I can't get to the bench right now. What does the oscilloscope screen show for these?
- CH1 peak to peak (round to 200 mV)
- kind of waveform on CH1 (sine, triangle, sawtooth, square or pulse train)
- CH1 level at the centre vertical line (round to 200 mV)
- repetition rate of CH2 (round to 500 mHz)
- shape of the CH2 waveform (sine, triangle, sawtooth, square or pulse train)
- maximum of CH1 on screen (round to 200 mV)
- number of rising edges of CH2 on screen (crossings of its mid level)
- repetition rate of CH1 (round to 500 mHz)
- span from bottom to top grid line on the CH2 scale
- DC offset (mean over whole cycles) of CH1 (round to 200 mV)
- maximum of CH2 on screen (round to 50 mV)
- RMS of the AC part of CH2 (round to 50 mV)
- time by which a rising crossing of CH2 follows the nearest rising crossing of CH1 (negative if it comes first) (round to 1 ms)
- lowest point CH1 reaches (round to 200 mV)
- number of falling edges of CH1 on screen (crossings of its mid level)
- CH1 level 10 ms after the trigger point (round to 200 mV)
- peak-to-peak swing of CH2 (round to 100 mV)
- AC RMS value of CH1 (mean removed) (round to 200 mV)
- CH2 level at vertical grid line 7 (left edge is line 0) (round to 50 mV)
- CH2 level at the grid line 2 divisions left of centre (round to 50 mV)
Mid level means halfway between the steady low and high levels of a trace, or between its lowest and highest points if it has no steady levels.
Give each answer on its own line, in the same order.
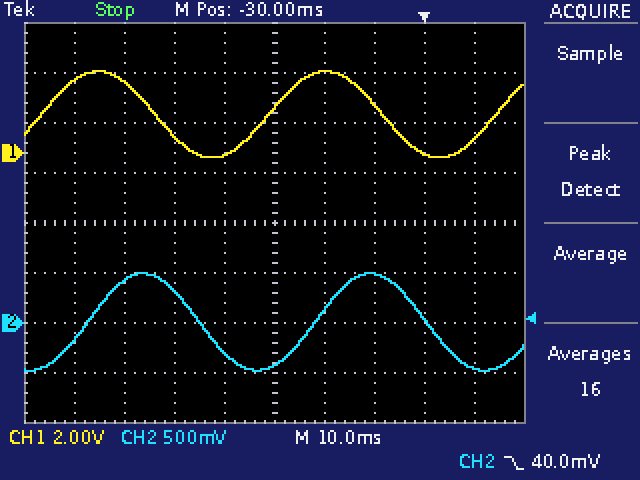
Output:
3.4 V
sine
1.8 V
22.0 Hz
sine
3.2 V
2
22.0 Hz
4 V
1.6 V
500 mV
350 mV
+9 ms
-200 mV
2
600 mV
1.00 V
1.2 V
500 mV
300 mV
